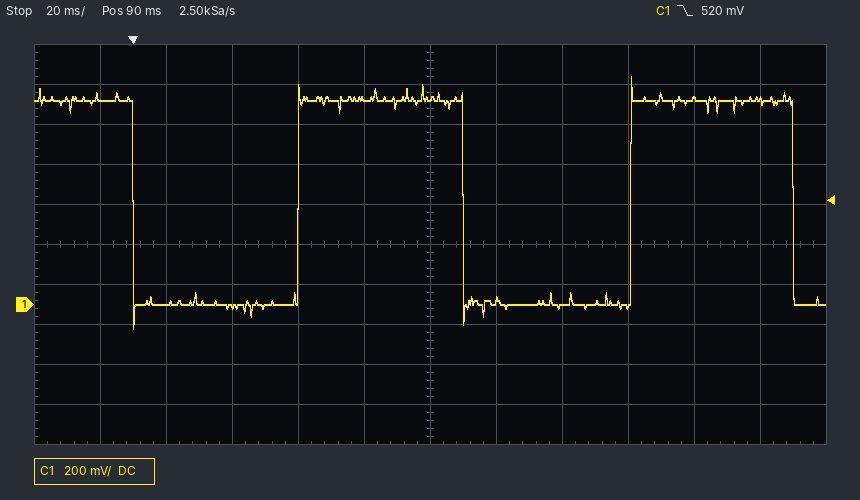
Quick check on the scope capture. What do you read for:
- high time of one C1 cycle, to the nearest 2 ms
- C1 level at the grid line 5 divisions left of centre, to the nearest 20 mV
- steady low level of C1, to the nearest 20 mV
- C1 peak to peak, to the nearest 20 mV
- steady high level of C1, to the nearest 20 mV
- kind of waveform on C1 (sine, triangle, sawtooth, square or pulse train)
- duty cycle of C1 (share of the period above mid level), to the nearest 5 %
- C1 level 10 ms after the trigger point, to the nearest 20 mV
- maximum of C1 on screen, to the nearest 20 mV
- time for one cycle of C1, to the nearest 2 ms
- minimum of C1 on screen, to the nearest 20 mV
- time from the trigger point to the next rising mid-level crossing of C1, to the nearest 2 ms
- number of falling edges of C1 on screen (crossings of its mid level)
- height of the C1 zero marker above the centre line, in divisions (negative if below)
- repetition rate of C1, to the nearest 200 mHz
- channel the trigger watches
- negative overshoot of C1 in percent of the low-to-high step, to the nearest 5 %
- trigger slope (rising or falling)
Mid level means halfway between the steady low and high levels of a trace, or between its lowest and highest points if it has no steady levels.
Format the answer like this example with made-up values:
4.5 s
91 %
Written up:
50 ms
1.04 V
0 mV
1.26 V
1.02 V
square
50 %
0 mV
1.14 V
100 ms
-120 mV
50 ms
3
-1.5 div
10.0 Hz
C1
10 %
falling
